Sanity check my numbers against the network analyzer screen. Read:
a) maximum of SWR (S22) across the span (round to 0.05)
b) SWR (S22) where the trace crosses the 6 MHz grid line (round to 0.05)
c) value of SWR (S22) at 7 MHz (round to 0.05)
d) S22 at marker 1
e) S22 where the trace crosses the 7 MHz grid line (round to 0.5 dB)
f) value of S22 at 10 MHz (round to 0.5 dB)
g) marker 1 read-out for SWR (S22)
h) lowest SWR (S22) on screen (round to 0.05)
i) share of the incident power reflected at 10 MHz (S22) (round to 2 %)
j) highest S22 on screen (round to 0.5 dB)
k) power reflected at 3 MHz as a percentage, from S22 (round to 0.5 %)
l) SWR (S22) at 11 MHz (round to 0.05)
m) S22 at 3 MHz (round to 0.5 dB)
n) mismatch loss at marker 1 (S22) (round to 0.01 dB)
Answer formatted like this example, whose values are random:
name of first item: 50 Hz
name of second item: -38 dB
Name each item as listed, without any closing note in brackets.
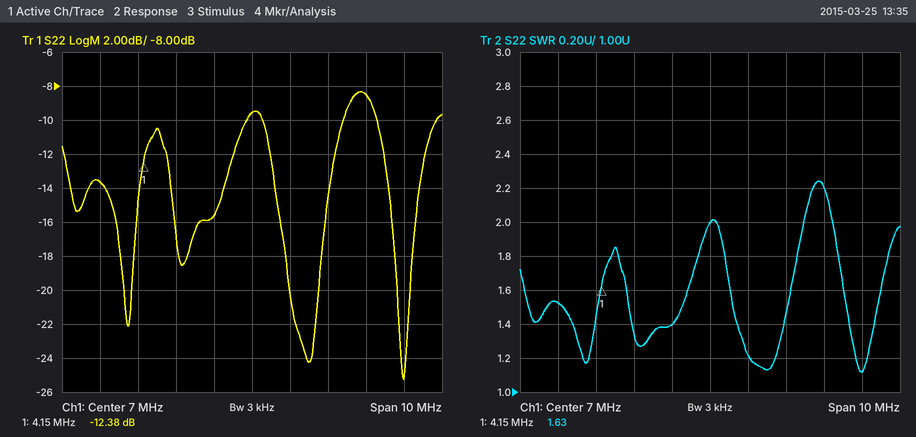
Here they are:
maximum of SWR (S22) across the span: 2.25
SWR (S22) where the trace crosses the 6 MHz grid line: 1.40
value of SWR (S22) at 7 MHz: 2.00
S22 at marker 1: -12.38 dB
S22 where the trace crosses the 7 MHz grid line: -9.5 dB
value of S22 at 10 MHz: -8.5 dB
marker 1 read-out for SWR: 1.63
lowest SWR (S22) on screen: 1.10
share of the incident power reflected at 10 MHz (S22): 14 %
highest S22 on screen: -8.5 dB
power reflected at 3 MHz as a percentage, from S22: 4.5 %
SWR (S22) at 11 MHz: 1.10
S22 at 3 MHz: -13.5 dB
mismatch loss at marker 1 (S22): 0.26 dB
